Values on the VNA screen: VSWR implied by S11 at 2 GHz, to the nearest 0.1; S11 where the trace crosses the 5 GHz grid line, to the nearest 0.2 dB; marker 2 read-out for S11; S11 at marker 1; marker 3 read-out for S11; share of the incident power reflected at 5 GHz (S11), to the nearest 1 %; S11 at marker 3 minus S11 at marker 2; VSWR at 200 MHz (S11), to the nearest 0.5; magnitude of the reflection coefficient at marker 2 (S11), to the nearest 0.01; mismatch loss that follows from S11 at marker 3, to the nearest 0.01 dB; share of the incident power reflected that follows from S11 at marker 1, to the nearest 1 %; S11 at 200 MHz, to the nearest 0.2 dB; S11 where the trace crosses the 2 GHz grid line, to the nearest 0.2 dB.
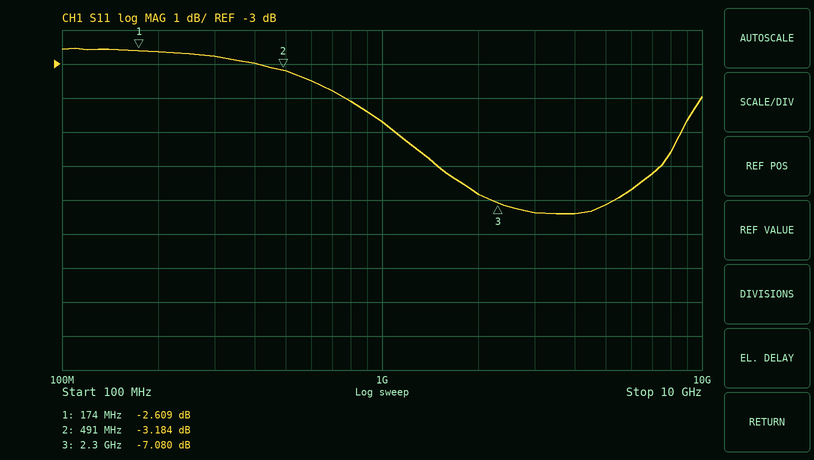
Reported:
2.7
-7.2 dB
-3.184 dB
-2.609 dB
-7.080 dB
19 %
-3.896 dB
6.5
0.69
0.95 dB
55 %
-2.6 dB
-6.8 dB
